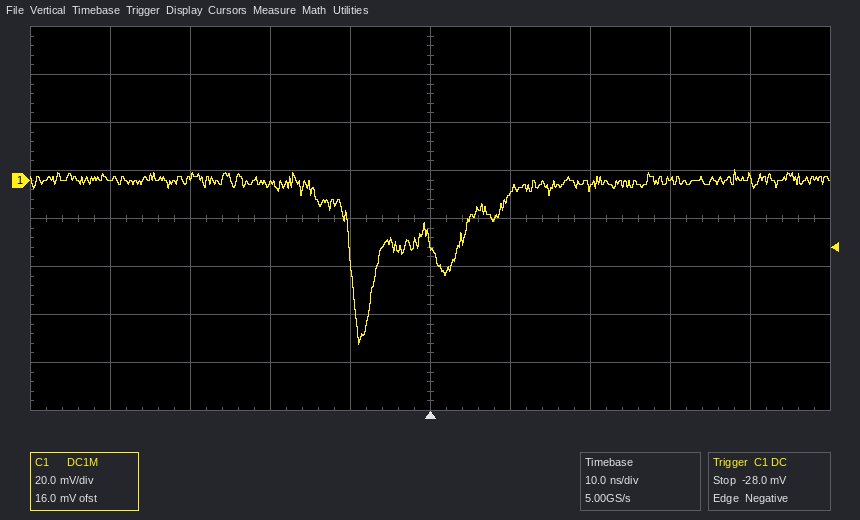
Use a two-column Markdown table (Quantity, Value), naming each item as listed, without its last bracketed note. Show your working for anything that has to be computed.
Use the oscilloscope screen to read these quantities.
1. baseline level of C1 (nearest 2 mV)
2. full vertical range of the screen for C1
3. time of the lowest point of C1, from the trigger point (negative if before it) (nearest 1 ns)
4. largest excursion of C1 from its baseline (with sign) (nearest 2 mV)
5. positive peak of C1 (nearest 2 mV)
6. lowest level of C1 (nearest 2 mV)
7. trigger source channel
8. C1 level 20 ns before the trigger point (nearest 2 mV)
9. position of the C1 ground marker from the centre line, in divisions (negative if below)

| Quantity | Value |
|---|---|
| baseline level of C1 | 0 mV |
| full vertical range of the screen for C1 | 160 mV |
| time of the lowest point of C1, from the trigger point (negative if before it) | -9 ns |
| largest excursion of C1 from its baseline (with sign) | -68 mV − (0 mV) = -68 mV |
| positive peak of C1 | 4 mV |
| lowest level of C1 | -68 mV |
| trigger source channel | C1 |
| C1 level 20 ns before the trigger point | -2 mV |
| position of the C1 ground marker from the centre line, in divisions | +0.8 div |
